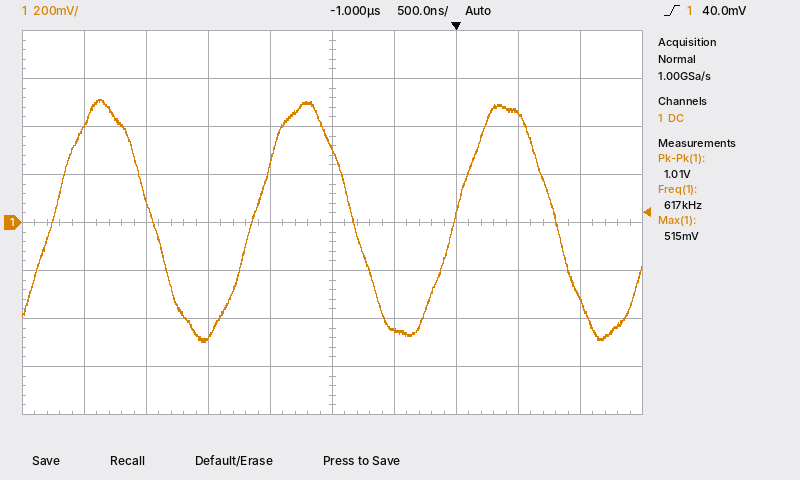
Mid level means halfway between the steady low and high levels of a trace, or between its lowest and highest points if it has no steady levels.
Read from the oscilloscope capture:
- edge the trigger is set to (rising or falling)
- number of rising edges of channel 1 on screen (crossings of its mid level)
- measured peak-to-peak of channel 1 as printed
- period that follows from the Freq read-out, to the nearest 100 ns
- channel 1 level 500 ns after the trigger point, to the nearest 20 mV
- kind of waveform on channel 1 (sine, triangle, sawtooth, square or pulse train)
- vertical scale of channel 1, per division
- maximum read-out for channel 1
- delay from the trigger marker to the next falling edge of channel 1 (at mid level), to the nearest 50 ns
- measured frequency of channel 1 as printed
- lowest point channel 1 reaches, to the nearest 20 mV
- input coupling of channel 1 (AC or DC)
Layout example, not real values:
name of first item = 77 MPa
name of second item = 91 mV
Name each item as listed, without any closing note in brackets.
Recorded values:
edge the trigger is set to = rising
number of rising edges of channel 1 on screen = 3
measured peak-to-peak of channel 1 as printed = 1.01 V
period that follows from the Freq read-out, to the nearest 100 ns = 1.6 µs
channel 1 level 500 ns after the trigger point, to the nearest 20 mV = 460 mV
kind of waveform on channel 1 = sine
vertical scale of channel 1, per division = 200 mV
maximum read-out for channel 1 = 515 mV
delay from the trigger marker to the next falling edge of channel 1 (at mid level), to the nearest 50 ns = 800 ns
measured frequency of channel 1 as printed = 617 kHz
lowest point channel 1 reaches, to the nearest 20 mV = -500 mV
input coupling of channel 1 = DC
